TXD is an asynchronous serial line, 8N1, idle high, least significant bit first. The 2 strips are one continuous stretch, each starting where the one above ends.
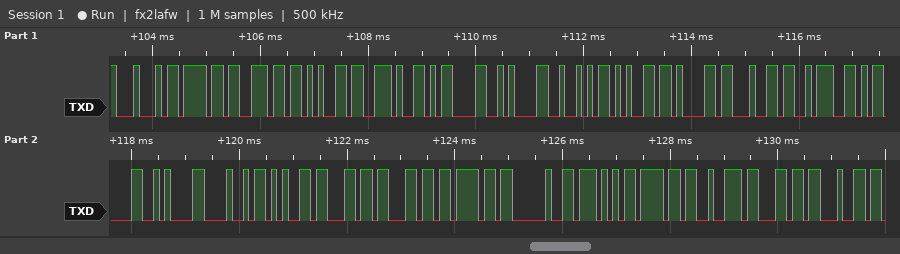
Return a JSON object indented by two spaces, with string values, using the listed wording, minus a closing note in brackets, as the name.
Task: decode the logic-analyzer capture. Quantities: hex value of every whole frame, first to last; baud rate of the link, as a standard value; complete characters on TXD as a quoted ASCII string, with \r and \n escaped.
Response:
{
  "hex value of every whole frame, first to last": "44 6F 6E 65 2E 0D 0A 52 65 61 64 3A 0D 0A 48 65 6C 6C 6F 20 57 6F 72 6C 64",
  "baud rate of the link, as a standard value": "9600 baud",
  "complete characters on TXD as a quoted ASCII string, with \\r and \\n escaped": "\"Done.\\r\\nRead:\\r\\nHello World\""
}
